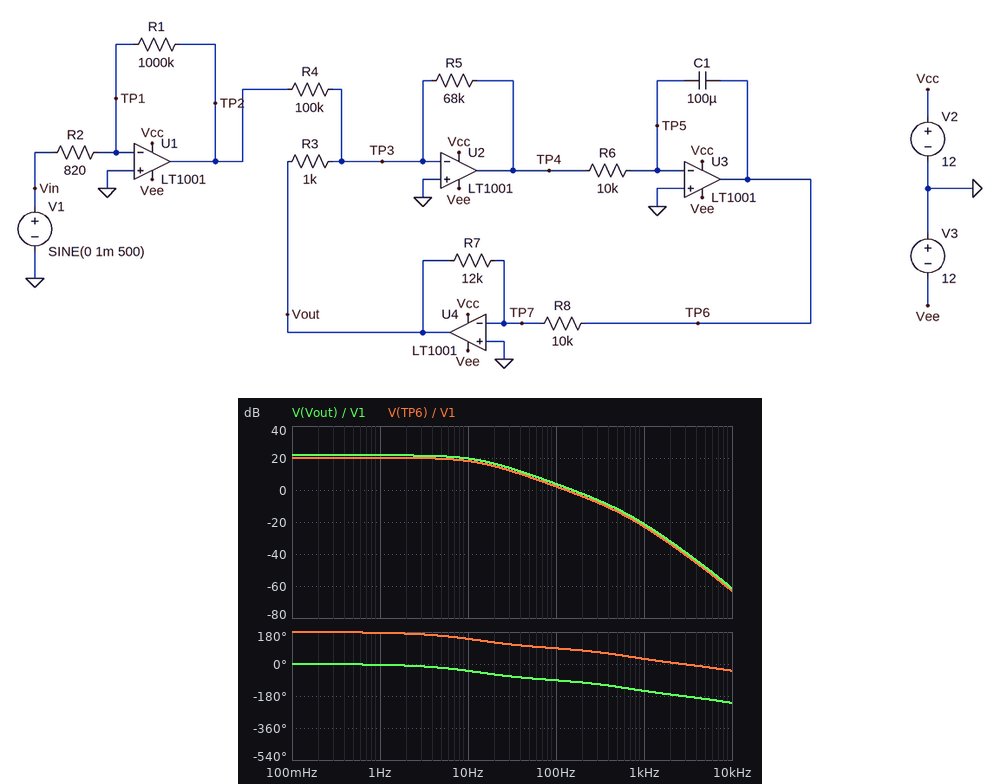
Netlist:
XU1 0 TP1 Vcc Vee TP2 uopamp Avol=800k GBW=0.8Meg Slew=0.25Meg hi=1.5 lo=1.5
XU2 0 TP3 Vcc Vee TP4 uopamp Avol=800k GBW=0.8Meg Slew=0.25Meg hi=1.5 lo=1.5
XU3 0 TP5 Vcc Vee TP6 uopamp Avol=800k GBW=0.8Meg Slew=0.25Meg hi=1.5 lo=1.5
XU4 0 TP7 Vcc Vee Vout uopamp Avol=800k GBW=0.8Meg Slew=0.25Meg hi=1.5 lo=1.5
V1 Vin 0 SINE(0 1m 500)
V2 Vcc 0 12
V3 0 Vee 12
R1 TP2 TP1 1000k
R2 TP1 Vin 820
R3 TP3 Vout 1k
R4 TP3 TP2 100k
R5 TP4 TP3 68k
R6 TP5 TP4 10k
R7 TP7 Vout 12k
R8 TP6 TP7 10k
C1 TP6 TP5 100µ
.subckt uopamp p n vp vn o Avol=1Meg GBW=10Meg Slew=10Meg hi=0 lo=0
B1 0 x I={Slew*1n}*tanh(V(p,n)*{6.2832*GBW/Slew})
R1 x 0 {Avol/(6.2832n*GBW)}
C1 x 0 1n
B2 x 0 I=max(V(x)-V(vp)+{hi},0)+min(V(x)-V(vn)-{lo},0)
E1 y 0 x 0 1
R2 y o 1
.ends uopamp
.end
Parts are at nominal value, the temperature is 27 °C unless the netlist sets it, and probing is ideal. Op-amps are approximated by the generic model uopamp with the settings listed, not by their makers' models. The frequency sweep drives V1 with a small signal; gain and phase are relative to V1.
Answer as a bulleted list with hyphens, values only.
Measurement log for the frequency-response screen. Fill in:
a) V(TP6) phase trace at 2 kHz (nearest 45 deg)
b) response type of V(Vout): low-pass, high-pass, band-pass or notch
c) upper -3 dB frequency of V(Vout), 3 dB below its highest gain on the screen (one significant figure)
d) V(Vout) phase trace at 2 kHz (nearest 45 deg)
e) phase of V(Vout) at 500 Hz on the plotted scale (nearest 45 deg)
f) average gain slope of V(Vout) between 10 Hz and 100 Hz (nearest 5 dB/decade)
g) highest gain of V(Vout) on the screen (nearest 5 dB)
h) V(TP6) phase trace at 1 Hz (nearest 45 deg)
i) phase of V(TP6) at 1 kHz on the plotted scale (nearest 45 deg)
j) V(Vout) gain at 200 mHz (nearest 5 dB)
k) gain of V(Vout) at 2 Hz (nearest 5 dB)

- 0 deg
- low-pass
- 10 Hz
- -180 deg
- -135 deg
- -15 dB/decade
- 20 dB
- 180 deg
- 45 deg
- 20 dB
- 20 dB
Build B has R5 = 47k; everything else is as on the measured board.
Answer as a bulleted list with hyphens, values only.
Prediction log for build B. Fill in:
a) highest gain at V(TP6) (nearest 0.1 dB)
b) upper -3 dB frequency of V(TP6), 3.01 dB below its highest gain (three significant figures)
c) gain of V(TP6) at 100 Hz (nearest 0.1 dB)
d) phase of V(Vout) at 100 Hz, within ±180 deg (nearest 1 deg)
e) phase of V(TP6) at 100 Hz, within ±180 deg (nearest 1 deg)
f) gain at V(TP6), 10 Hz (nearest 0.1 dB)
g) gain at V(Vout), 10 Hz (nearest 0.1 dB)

- 20.1 dB
- 8.98 Hz
- -0.9 dB
- -94 deg
- 86 deg
- 16.6 dB
- 18.2 dB
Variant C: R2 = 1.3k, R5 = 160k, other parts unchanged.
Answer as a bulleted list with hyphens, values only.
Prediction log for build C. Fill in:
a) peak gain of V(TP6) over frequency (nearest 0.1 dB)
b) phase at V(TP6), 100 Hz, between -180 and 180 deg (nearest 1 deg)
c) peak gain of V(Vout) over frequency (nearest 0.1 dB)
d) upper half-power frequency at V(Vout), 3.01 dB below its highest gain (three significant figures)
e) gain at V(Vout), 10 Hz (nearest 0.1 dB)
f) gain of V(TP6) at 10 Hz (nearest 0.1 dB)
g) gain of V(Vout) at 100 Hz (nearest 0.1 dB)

- 16.1 dB
- 100 deg
- 17.7 dB
- 30.7 Hz
- 17.3 dB
- 15.7 dB
- 7.0 dB
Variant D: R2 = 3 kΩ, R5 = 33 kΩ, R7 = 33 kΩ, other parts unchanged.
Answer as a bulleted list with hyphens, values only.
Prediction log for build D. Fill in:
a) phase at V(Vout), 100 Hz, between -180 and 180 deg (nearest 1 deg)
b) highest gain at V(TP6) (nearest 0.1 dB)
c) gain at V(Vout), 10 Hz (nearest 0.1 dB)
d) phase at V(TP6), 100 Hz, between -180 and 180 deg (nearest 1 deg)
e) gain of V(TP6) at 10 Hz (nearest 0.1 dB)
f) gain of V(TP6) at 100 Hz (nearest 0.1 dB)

- -83 deg
- 0.1 dB
- 9.2 dB
- 97 deg
- -1.2 dB
- -15.3 dB
